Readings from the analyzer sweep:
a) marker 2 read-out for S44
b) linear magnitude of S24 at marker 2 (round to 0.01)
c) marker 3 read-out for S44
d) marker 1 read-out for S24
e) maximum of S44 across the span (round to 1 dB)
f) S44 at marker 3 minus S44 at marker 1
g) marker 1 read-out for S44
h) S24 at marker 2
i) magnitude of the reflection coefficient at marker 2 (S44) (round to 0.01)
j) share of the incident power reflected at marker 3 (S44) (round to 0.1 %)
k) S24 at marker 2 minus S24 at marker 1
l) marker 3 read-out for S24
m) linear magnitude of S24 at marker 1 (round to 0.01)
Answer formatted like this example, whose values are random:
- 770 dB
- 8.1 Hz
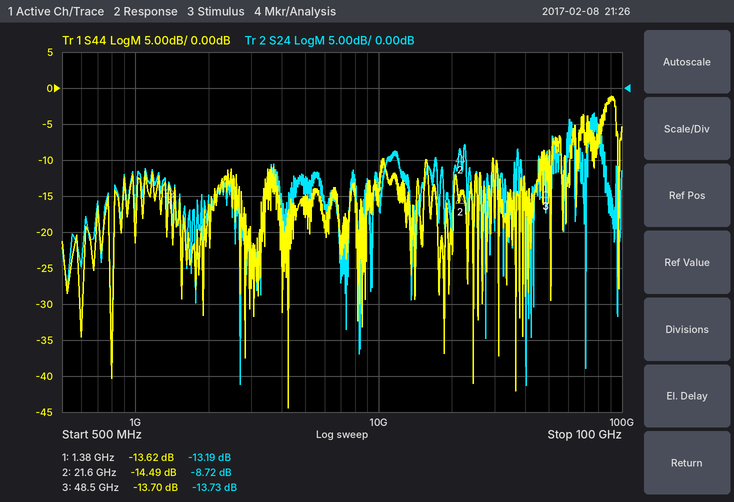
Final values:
- -14.49 dB
- 0.37
- -13.70 dB
- -13.19 dB
- -1 dB
- -0.08 dB
- -13.62 dB
- -8.72 dB
- 0.19
- 4.3 %
- 4.47 dB
- -13.73 dB
- 0.22
